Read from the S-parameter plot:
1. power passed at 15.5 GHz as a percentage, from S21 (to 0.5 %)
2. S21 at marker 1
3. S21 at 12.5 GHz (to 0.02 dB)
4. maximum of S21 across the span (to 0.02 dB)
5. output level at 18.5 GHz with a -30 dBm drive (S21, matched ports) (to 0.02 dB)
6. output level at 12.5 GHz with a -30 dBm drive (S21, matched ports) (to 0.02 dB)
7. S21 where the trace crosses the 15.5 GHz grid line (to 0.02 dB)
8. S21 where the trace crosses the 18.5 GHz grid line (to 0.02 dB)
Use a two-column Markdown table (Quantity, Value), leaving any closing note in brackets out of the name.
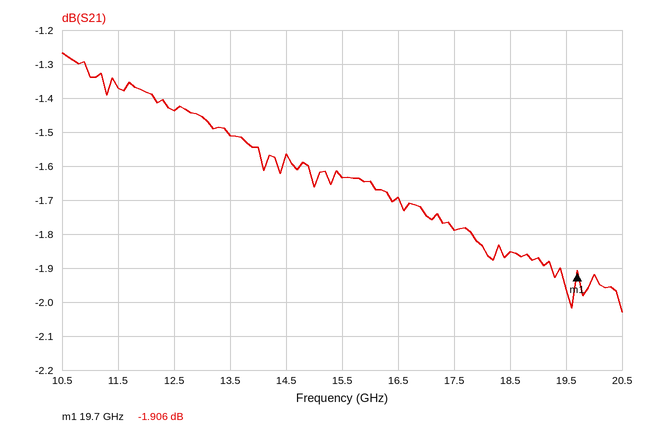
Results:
| Quantity | Value |
|---|---|
| power passed at 15.5 GHz as a percentage, from S21 | 68.5 % |
| S21 at marker 1 | -1.906 dB |
| S21 at 12.5 GHz | -1.44 dB |
| maximum of S21 across the span | -1.26 dB |
| output level at 18.5 GHz with a -30 dBm drive (S21, matched ports) | -31.86 dBm |
| output level at 12.5 GHz with a -30 dBm drive (S21, matched ports) | -31.44 dBm |
| S21 where the trace crosses the 15.5 GHz grid line | -1.64 dB |
| S21 where the trace crosses the 18.5 GHz grid line | -1.86 dB |
